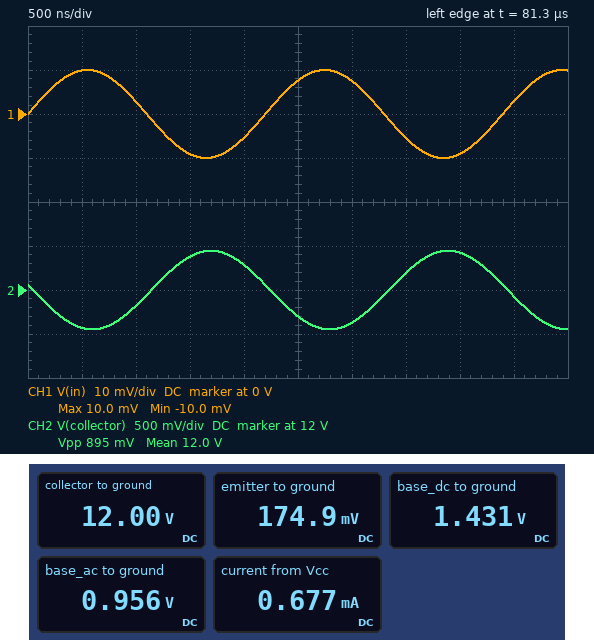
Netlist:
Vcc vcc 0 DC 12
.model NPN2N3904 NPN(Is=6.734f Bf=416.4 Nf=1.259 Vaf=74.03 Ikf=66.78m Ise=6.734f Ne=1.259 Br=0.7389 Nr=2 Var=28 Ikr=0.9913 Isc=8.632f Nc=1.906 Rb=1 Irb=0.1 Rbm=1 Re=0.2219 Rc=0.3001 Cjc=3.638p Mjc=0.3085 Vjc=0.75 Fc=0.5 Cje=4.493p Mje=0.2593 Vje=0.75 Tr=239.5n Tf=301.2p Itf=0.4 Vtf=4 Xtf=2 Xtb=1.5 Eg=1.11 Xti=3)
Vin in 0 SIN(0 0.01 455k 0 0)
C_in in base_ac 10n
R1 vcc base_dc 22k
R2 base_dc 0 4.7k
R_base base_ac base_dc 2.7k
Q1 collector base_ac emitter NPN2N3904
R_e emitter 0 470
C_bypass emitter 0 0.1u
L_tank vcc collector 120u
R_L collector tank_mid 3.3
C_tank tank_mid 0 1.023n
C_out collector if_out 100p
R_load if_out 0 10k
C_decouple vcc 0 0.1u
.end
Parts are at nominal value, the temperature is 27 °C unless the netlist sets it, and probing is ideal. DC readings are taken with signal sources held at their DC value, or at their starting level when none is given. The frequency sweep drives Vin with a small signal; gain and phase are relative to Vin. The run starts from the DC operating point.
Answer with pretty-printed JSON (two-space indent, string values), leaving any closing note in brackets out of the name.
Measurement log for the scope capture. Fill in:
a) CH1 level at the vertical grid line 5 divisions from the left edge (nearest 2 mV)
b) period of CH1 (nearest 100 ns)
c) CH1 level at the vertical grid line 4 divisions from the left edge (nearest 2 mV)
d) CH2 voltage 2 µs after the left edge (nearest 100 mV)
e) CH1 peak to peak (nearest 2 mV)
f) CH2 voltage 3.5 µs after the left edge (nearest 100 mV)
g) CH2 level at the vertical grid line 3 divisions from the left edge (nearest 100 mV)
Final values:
{
  "CH1 level at the vertical grid line 5 divisions from the left edge": "8 mV",
  "period of CH1": "2.2 µs",
  "CH1 level at the vertical grid line 4 divisions from the left edge": "-6 mV",
  "CH2 voltage 2 µs after the left edge": "12.3 V",
  "CH1 peak to peak": "20 mV",
  "CH2 voltage 3.5 µs after the left edge": "12.2 V",
  "CH2 level at the vertical grid line 3 divisions from the left edge": "12.4 V"
}
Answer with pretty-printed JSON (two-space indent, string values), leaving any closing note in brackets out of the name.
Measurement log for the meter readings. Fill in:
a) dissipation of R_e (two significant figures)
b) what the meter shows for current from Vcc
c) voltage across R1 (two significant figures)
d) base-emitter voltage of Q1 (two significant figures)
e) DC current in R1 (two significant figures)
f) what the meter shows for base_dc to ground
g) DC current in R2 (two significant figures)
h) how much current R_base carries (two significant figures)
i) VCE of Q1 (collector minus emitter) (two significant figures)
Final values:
{
  "dissipation of R_e": "65 µW",
  "what the meter shows for current from Vcc": "0.677 mA",
  "voltage across R1": "11 V",
  "base-emitter voltage of Q1": "780 mV",
  "DC current in R1": "480 µA",
  "what the meter shows for base_dc to ground": "1.431 V",
  "DC current in R2": "300 µA",
  "how much current R_base carries": "180 µA",
  "VCE of Q1 (collector minus emitter)": "12 V"
}
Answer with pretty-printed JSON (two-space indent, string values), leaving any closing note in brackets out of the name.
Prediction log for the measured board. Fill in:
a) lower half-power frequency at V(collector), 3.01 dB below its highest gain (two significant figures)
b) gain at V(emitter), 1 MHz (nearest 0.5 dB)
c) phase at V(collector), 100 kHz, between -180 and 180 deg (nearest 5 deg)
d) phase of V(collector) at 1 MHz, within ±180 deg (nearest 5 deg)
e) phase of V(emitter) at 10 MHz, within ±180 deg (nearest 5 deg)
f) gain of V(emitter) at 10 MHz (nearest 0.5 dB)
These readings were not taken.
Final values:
{
  "lower half-power frequency at V(collector), 3.01 dB below its highest gain": "440 kHz",
  "gain at V(emitter), 1 MHz": "-35.0 dB",
  "phase at V(collector), 100 kHz, between -180 and 180 deg": "-45 deg",
  "phase of V(collector) at 1 MHz, within ±180 deg": "100 deg",
  "phase of V(emitter) at 10 MHz, within ±180 deg": "-85 deg",
  "gain of V(emitter) at 10 MHz": "-55.0 dB"
}
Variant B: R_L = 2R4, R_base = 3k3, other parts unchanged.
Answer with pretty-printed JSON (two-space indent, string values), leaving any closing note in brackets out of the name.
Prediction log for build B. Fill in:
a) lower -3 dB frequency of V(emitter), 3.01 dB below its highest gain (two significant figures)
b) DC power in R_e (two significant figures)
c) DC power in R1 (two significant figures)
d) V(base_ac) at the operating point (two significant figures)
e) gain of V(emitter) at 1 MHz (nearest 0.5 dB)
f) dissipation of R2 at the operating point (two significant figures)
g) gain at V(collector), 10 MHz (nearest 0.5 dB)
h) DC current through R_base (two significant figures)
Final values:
{
  "lower -3 dB frequency of V(emitter), 3.01 dB below its highest gain": "3.0 kHz",
  "DC power in R_e": "56 µW",
  "DC power in R1": "5.0 mW",
  "V(base_ac) at the operating point": "940 mV",
  "gain of V(emitter) at 1 MHz": "-35.5 dB",
  "dissipation of R2 at the operating point": "470 µW",
  "gain at V(collector), 10 MHz": "-21.0 dB",
  "DC current through R_base": "160 µA"
}
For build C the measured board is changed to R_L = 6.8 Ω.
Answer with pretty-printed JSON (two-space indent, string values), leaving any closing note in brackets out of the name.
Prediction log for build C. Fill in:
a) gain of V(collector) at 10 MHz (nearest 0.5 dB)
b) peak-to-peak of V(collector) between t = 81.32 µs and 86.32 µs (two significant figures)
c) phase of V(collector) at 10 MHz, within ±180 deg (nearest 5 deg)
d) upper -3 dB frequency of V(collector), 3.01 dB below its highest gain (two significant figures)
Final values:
{
  "gain of V(collector) at 10 MHz": "-20.0 dB",
  "peak-to-peak of V(collector) between t = 81.32 µs and 86.32 µs": "730 mV",
  "phase of V(collector) at 10 MHz, within ±180 deg": "115 deg",
  "upper -3 dB frequency of V(collector), 3.01 dB below its highest gain": "460 kHz"
}
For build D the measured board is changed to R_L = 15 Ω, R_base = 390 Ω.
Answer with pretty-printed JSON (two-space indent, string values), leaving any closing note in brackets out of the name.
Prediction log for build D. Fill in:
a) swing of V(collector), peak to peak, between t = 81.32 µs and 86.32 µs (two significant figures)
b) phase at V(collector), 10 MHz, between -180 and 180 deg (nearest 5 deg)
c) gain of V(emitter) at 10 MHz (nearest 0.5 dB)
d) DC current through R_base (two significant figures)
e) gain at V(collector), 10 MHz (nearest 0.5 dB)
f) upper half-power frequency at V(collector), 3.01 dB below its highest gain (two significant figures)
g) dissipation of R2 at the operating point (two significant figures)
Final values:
{
  "swing of V(collector), peak to peak, between t = 81.32 µs and 86.32 µs": "700 mV",
  "phase at V(collector), 10 MHz, between -180 and 180 deg": "135 deg",
  "gain of V(emitter) at 10 MHz": "-52.0 dB",
  "DC current through R_base": "250 µA",
  "gain at V(collector), 10 MHz": "-15.0 dB",
  "upper half-power frequency at V(collector), 3.01 dB below its highest gain": "470 kHz",
  "dissipation of R2 at the operating point": "280 µW"
}
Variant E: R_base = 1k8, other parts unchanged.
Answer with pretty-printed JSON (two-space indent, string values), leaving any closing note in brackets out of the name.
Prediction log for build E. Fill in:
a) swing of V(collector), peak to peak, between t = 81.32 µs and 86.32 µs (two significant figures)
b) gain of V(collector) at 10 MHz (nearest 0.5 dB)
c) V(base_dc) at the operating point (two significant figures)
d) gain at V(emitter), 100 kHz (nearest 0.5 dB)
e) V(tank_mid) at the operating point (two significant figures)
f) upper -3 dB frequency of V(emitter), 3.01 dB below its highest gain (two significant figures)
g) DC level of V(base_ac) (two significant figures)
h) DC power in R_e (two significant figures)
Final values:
{
  "swing of V(collector), peak to peak, between t = 81.32 µs and 86.32 µs": "1.0 V",
  "gain of V(collector) at 10 MHz": "-19.5 dB",
  "V(base_dc) at the operating point": "1.3 V",
  "gain at V(emitter), 100 kHz": "-17.5 dB",
  "V(tank_mid) at the operating point": "12 V",
  "upper -3 dB frequency of V(emitter), 3.01 dB below its highest gain": "130 kHz",
  "DC level of V(base_ac)": "980 mV",
  "DC power in R_e": "83 µW"
}
